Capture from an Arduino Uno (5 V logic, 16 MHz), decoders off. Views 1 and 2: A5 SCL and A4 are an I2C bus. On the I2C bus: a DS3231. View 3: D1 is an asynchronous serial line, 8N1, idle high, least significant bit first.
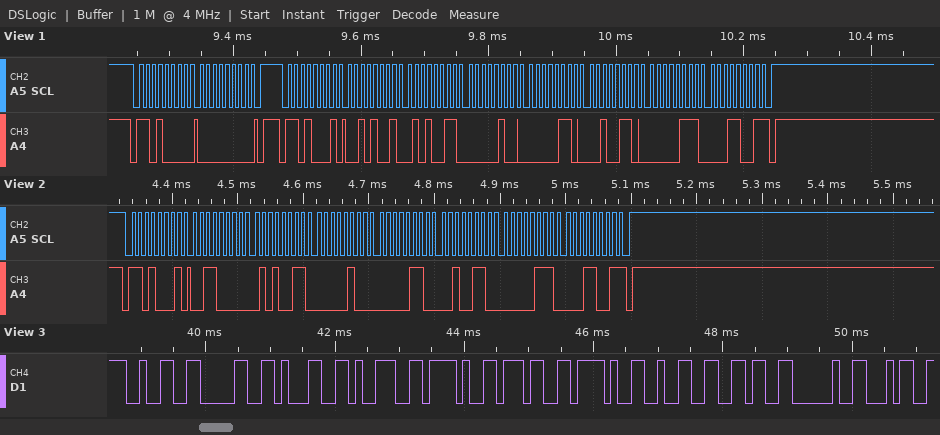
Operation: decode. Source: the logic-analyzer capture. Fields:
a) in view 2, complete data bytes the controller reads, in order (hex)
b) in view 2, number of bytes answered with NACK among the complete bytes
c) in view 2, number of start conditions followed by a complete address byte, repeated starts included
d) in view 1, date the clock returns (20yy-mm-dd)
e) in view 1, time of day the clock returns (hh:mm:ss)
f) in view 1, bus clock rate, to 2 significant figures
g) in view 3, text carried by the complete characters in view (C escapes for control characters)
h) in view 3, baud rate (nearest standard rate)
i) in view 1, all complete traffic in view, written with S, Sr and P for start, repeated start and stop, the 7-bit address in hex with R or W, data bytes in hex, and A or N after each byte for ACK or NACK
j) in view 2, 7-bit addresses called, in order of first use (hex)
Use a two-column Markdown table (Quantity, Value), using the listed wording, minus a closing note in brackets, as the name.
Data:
| Quantity | Value |
|---|---|
| in view 2, complete data bytes the controller reads, in order | 30 53 04 06 26 07 19 |
| in view 2, number of bytes answered with NACK among the complete bytes | 1 |
| in view 2, number of start conditions followed by a complete address byte, repeated starts included | 1 |
| in view 1, date the clock returns | 2019-07-26 |
| in view 1, time of day the clock returns | 04:53:29 |
| in view 1, bus clock rate, to 2 significant figures | 100 kHz |
| in view 3, text carried by the complete characters in view | "2019/7/26 4" |
| in view 3, baud rate | 9600 baud |
| in view 1, all complete traffic in view, written with S, Sr and P for start, repeated start and stop, the 7-bit address in hex with R or W, data bytes in hex, and A or N after each byte for ACK or NACK | S 68W A 00 A P S 68R A 29 A 53 A 04 A 06 A 26 A 07 A 19 N P |
| in view 2, 7-bit addresses called, in order of first use | 0x68 |
